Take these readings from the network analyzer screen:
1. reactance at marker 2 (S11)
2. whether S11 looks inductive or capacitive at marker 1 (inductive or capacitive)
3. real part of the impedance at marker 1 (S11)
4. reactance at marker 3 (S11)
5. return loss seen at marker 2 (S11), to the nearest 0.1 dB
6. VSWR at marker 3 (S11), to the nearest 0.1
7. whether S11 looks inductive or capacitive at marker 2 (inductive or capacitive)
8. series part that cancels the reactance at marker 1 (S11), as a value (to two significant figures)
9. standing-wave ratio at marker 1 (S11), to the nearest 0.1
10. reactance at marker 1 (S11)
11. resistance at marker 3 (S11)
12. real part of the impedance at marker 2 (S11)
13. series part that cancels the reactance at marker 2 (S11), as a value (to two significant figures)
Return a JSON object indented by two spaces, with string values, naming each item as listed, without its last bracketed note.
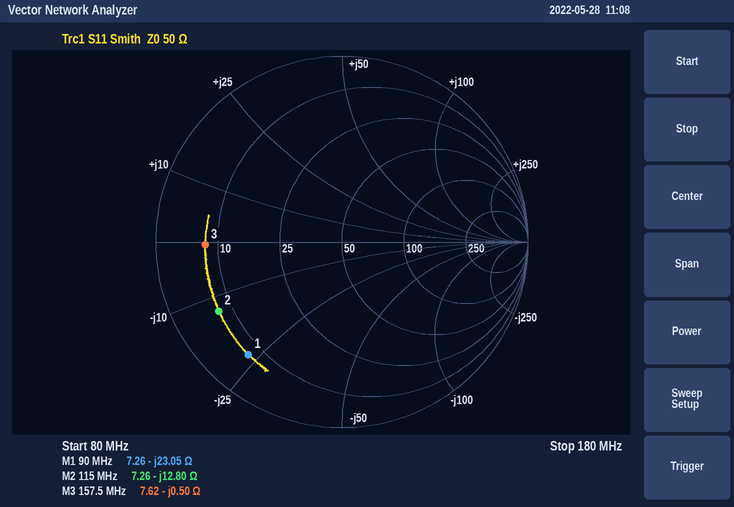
{
  "reactance at marker 2": "-12.80 Ω",
  "whether S11 looks inductive or capacitive at marker 1": "capacitive",
  "real part of the impedance at marker 1": "7.26 Ω",
  "reactance at marker 3": "-0.50 Ω",
  "return loss seen at marker 2 (S11), to the nearest 0.1 dB": "2.4 dB",
  "VSWR at marker 3 (S11), to the nearest 0.1": "6.6",
  "whether S11 looks inductive or capacitive at marker 2": "capacitive",
  "series part that cancels the reactance at marker 1 (S11), as a value": "41 nH",
  "standing-wave ratio at marker 1 (S11), to the nearest 0.1": "8.4",
  "reactance at marker 1": "-23.05 Ω",
  "resistance at marker 3": "7.62 Ω",
  "real part of the impedance at marker 2": "7.26 Ω",
  "series part that cancels the reactance at marker 2 (S11), as a value": "18 nH"
}
